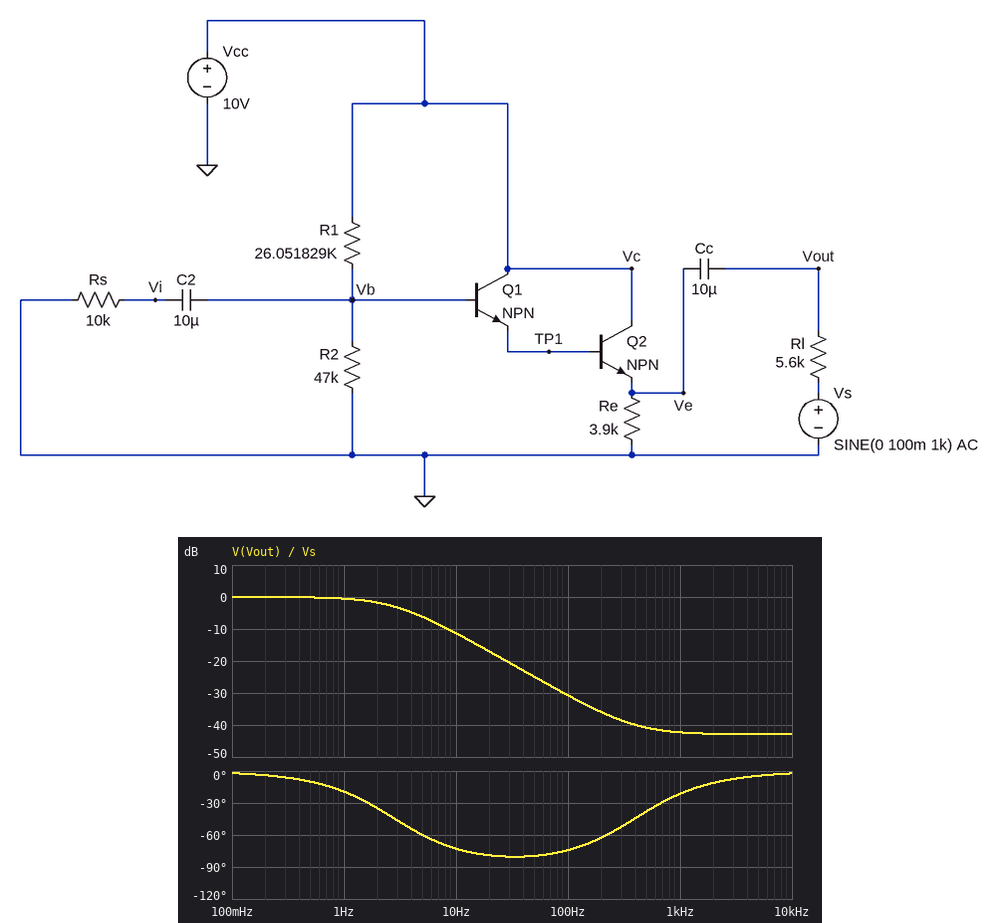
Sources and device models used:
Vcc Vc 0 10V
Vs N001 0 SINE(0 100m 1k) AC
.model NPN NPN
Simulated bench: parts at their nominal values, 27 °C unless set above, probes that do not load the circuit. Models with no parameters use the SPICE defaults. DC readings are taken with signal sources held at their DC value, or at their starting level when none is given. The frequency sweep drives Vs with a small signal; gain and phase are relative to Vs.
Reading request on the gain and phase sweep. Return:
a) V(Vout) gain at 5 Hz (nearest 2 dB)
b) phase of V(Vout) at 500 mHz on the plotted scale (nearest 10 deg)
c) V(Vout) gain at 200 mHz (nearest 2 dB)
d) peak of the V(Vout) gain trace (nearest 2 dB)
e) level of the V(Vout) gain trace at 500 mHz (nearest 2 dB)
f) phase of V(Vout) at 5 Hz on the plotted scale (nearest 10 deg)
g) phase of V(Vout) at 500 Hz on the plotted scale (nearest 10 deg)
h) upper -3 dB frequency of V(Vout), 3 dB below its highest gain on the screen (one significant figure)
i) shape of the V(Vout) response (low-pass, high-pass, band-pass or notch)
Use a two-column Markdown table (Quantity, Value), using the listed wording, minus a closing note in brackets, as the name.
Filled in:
| Quantity | Value |
|---|---|
| V(Vout) gain at 5 Hz | -6 dB |
| phase of V(Vout) at 500 mHz on the plotted scale | -10 deg |
| V(Vout) gain at 200 mHz | 0 dB |
| peak of the V(Vout) gain trace | 0 dB |
| level of the V(Vout) gain trace at 500 mHz | 0 dB |
| phase of V(Vout) at 5 Hz on the plotted scale | -60 deg |
| phase of V(Vout) at 500 Hz on the plotted scale | -40 deg |
| upper -3 dB frequency of V(Vout), 3 dB below its highest gain on the screen | 3 Hz |
| shape of the V(Vout) response | low-pass |
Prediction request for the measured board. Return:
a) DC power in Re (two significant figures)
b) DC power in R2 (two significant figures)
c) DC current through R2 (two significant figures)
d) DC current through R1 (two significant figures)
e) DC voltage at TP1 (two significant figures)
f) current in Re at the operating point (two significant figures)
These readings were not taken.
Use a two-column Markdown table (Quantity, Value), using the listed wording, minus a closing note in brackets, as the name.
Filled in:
| Quantity | Value |
|---|---|
| DC power in Re | 6.4 mW |
| DC power in R2 | 880 µW |
| DC current through R2 | 140 µA |
| DC current through R1 | 140 µA |
| DC voltage at TP1 | 5.8 V |
| current in Re at the operating point | 1.3 mA |
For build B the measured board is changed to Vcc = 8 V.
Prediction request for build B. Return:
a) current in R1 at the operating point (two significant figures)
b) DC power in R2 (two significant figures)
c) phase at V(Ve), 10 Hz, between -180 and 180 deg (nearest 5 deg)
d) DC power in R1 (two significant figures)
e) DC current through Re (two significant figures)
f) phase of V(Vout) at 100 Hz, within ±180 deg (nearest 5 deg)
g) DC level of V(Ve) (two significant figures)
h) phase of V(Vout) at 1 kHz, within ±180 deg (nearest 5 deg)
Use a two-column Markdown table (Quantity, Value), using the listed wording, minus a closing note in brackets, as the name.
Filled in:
| Quantity | Value |
|---|---|
| current in R1 at the operating point | 110 µA |
| DC power in R2 | 560 µW |
| phase at V(Ve), 10 Hz, between -180 and 180 deg | 15 deg |
| DC power in R1 | 310 µW |
| DC current through Re | 950 µA |
| phase of V(Vout) at 100 Hz, within ±180 deg | -70 deg |
| DC level of V(Ve) | 3.7 V |
| phase of V(Vout) at 1 kHz, within ±180 deg | -15 deg |
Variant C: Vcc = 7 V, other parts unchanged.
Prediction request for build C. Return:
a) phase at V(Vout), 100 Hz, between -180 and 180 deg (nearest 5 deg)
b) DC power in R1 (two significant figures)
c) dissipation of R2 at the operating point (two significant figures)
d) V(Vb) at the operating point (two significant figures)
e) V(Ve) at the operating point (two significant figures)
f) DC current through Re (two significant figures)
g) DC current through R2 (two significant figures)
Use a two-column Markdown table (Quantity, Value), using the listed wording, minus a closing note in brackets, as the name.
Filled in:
| Quantity | Value |
|---|---|
| phase at V(Vout), 100 Hz, between -180 and 180 deg | -65 deg |
| DC power in R1 | 240 µW |
| dissipation of R2 at the operating point | 430 µW |
| V(Vb) at the operating point | 4.5 V |
| V(Ve) at the operating point | 3.1 V |
| DC current through Re | 790 µA |
| DC current through R2 | 96 µA |
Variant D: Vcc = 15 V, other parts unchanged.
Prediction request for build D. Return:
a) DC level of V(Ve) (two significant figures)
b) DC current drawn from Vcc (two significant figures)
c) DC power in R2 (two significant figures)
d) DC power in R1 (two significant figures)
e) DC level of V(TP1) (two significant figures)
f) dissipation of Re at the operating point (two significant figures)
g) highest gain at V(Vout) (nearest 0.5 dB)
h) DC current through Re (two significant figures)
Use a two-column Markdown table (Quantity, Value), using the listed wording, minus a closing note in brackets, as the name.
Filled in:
| Quantity | Value |
|---|---|
| DC level of V(Ve) | 8.2 V |
| DC current drawn from Vcc | 2.3 mA |
| DC power in R2 | 2.0 mW |
| DC power in R1 | 1.1 mW |
| DC level of V(TP1) | 9.0 V |
| dissipation of Re at the operating point | 17 mW |
| highest gain at V(Vout) | 0 dB |
| DC current through Re | 2.1 mA |
